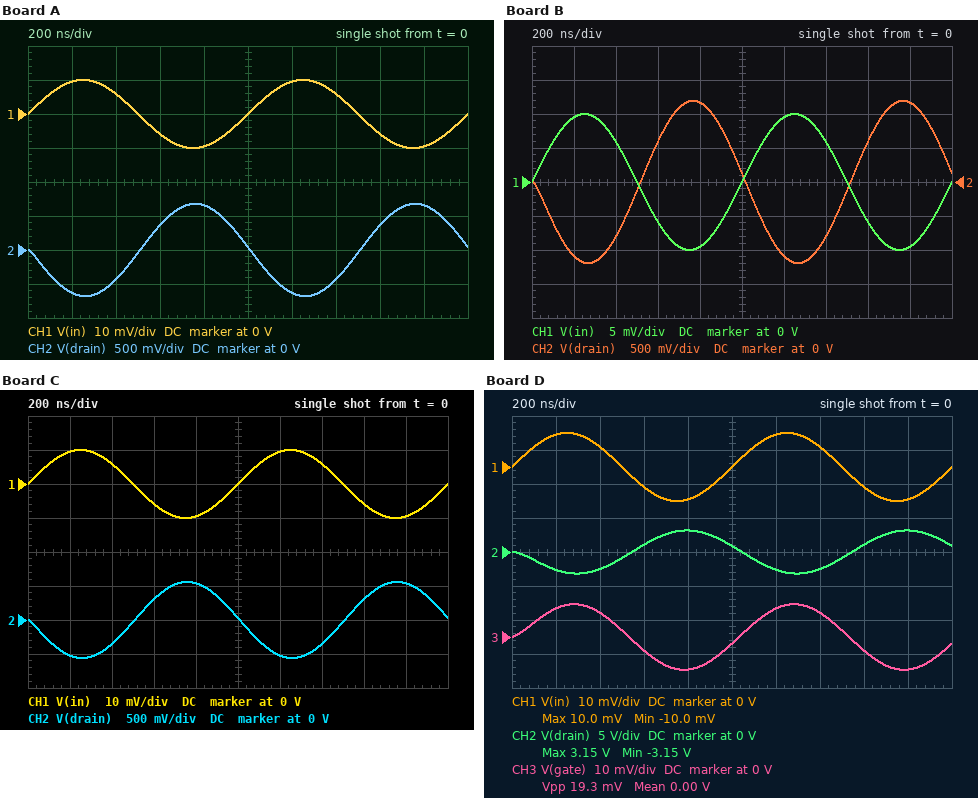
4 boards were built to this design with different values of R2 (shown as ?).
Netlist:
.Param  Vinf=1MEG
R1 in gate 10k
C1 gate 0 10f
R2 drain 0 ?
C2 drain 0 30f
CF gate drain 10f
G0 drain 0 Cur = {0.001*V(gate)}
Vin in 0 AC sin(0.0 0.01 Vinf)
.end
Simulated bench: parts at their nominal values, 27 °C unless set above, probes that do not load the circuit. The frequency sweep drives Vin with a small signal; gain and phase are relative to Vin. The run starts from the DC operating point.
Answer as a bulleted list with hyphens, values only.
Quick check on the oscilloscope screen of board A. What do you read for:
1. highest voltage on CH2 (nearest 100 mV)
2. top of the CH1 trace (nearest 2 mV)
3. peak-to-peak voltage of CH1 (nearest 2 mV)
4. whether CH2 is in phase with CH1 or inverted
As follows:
- 700 mV
- 10 mV
- 20 mV
- inverted
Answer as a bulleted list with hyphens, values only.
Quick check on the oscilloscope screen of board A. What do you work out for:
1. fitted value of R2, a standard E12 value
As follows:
- 68 kΩ
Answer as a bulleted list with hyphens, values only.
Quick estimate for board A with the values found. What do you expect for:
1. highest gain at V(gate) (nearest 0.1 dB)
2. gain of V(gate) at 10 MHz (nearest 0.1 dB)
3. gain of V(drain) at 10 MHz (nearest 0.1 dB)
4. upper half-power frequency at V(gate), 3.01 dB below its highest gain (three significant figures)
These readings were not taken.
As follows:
- 0 dB
- -1.2 dB
- 35.3 dB
- 17.9 MHz
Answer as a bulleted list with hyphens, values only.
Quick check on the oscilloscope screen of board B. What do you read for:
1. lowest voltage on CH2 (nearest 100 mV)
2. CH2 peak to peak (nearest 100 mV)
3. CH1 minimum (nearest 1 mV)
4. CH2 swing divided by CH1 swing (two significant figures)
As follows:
- -1.2 V
- 2.4 V
- -10 mV
- 120
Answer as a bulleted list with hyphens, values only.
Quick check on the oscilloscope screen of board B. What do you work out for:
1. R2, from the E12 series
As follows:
- 120 kΩ
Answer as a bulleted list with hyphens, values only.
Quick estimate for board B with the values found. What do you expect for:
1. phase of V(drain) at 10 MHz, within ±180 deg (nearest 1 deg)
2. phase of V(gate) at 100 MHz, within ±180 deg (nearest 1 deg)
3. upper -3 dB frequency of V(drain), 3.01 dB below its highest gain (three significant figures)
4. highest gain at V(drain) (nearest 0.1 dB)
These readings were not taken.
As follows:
- 133 deg
- -15 deg
- 9.39 MHz
- 41.6 dB
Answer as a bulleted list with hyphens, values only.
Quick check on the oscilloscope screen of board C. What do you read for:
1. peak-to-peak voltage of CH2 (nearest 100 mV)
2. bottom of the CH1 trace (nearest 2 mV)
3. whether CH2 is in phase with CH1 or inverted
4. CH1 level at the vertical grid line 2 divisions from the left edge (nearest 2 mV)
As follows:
- 1.1 V
- -10 mV
- inverted
- 6 mV
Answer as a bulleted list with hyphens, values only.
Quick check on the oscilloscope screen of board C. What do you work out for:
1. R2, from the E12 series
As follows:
- 56 kΩ
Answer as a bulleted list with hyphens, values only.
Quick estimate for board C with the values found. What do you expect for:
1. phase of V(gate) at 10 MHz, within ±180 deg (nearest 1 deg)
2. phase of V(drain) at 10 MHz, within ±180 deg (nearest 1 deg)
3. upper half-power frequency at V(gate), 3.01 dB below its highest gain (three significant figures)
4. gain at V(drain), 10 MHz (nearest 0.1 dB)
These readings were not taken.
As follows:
- -19 deg
- 153 deg
- 21.7 MHz
- 34.0 dB
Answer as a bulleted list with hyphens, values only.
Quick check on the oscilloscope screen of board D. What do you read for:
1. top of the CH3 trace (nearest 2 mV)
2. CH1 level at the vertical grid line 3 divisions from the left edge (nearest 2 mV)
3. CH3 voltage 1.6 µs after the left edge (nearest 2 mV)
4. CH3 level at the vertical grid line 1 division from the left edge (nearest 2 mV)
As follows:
- 10 mV
- -6 mV
- -4 mV
- 8 mV
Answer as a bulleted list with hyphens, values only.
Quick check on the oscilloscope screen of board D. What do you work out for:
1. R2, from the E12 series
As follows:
- 330 kΩ
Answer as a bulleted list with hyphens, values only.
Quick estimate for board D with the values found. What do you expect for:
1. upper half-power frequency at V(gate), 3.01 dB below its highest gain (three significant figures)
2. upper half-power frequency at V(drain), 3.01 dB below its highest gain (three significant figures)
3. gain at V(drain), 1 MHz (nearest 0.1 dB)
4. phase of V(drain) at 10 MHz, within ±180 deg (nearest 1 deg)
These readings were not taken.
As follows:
- 3.75 MHz
- 3.43 MHz
- 50.0 dB
- 109 deg
